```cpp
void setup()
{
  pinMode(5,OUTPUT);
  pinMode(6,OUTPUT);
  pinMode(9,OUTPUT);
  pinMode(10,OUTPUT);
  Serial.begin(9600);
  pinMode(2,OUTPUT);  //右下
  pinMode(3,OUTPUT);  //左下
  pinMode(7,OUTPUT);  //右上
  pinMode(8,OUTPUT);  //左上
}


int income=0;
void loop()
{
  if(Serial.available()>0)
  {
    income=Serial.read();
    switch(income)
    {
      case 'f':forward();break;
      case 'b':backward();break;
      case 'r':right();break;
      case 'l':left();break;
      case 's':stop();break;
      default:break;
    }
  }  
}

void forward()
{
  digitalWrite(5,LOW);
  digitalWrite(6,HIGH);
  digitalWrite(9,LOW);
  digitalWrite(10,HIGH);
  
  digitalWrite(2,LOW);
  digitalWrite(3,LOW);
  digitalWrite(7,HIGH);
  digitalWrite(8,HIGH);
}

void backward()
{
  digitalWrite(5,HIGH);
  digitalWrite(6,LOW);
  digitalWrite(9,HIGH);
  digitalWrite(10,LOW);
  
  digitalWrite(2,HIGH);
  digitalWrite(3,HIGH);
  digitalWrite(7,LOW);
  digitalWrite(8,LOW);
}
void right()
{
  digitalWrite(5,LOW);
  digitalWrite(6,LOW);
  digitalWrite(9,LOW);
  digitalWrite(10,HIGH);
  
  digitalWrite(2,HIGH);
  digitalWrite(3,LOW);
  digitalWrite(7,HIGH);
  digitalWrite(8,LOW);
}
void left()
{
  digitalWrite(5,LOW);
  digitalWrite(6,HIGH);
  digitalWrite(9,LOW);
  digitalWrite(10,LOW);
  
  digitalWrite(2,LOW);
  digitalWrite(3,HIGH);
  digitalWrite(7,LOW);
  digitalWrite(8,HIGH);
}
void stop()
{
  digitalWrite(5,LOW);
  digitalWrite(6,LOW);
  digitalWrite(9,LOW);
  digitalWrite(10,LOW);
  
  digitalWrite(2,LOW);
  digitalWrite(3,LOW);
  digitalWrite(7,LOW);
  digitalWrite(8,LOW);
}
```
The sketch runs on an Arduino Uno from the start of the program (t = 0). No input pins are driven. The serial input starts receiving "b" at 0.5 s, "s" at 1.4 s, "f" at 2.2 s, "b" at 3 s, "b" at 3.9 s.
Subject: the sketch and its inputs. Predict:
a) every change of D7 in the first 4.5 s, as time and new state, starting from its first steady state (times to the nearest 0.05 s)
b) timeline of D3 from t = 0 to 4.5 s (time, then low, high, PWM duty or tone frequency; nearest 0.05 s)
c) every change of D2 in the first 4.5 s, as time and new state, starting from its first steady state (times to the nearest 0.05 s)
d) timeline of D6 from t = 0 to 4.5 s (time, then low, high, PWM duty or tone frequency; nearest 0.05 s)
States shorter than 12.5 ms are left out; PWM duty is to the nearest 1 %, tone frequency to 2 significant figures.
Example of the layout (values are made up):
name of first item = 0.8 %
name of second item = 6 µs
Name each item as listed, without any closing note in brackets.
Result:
every change of D7 in the first 4.5 s, as time and new state, starting from its first steady state = 0 s low; 2.2 s high; 3 s low
timeline of D3 from t = 0 to 4.5 s = 0 s low; 0.5 s high; 1.4 s low; 3 s high
every change of D2 in the first 4.5 s, as time and new state, starting from its first steady state = 0 s low; 0.5 s high; 1.4 s low; 3 s high
timeline of D6 from t = 0 to 4.5 s = 0 s low; 2.2 s high; 3 s low
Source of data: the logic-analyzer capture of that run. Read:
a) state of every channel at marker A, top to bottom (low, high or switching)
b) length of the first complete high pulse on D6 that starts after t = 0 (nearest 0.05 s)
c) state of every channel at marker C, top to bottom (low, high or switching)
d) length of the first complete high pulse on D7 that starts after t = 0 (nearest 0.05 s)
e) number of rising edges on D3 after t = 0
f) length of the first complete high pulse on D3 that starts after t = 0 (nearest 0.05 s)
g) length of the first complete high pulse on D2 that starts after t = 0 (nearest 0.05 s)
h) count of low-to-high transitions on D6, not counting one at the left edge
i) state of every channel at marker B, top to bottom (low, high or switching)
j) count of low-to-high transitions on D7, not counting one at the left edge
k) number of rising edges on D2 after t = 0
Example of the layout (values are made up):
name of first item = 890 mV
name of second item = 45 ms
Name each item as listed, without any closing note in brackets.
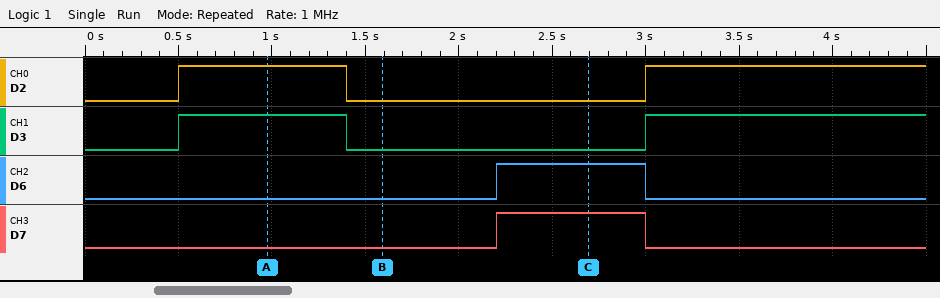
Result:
state of every channel at marker A, top to bottom = D2 high, D3 high, D6 low, D7 low
length of the first complete high pulse on D6 that starts after t = 0 = 0.80 s
state of every channel at marker C, top to bottom = D2 low, D3 low, D6 high, D7 high
length of the first complete high pulse on D7 that starts after t = 0 = 0.80 s
number of rising edges on D3 after t = 0 = 2
length of the first complete high pulse on D3 that starts after t = 0 = 0.90 s
length of the first complete high pulse on D2 that starts after t = 0 = 0.90 s
count of low-to-high transitions on D6, not counting one at the left edge = 1
state of every channel at marker B, top to bottom = D2 low, D3 low, D6 low, D7 low
count of low-to-high transitions on D7, not counting one at the left edge = 1
number of rising edges on D2 after t = 0 = 2
